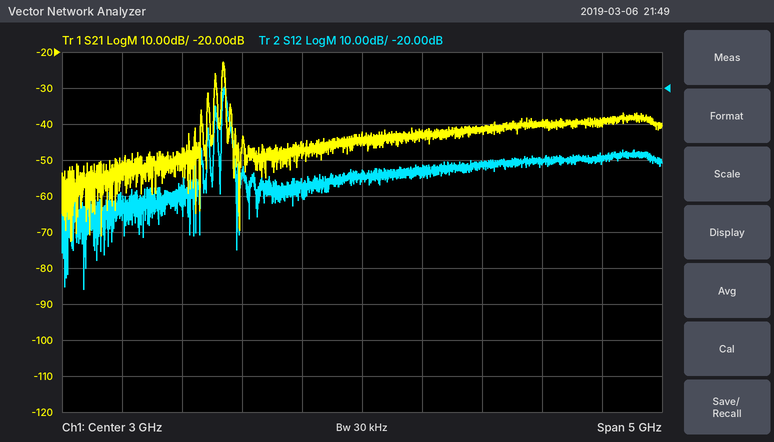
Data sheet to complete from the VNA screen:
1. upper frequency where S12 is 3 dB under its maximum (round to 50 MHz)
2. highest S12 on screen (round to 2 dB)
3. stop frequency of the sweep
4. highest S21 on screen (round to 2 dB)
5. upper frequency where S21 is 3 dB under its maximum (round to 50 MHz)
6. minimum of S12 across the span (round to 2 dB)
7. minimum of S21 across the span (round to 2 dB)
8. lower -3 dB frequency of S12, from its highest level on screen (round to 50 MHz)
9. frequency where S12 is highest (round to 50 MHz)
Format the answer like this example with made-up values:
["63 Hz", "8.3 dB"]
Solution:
["1.85 GHz", "-20 dB", "5.5 GHz", "-22 dB", "1.85 GHz", "-76 dB", "-72 dB", "1.85 GHz", "1.85 GHz"]
